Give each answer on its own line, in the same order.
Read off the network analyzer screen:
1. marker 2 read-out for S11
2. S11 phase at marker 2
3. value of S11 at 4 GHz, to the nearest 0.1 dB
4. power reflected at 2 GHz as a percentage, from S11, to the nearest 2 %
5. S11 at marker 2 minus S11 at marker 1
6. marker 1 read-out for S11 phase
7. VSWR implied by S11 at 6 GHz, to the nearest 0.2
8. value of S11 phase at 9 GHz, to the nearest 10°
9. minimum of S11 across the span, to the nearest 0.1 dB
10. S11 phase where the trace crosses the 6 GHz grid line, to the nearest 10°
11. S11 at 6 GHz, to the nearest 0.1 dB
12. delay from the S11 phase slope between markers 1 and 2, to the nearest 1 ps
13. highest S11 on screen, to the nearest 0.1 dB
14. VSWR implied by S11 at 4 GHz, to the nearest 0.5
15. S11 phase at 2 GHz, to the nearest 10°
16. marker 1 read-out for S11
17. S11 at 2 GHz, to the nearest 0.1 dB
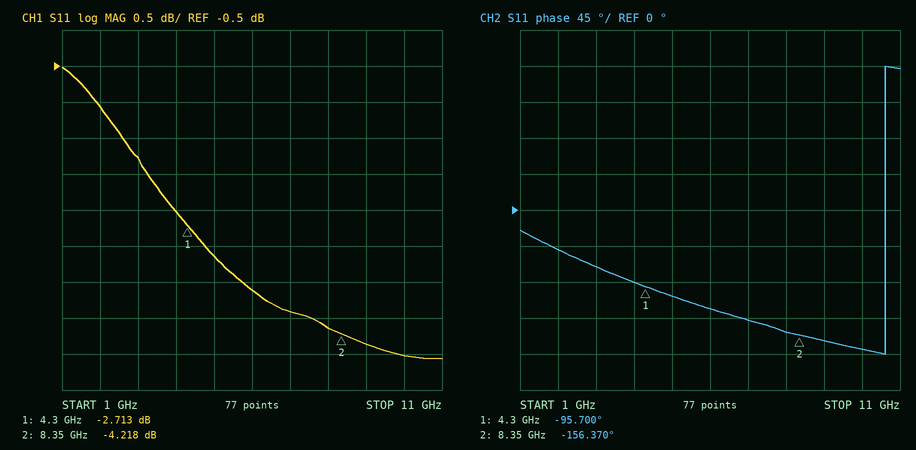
-4.218 dB
-156.370°
-2.5 dB
78 %
-1.505 dB
-95.700°
4.8
-160°
-4.6 dB
-120°
-3.6 dB
42 ps
-0.5 dB
7.0
-50°
-2.713 dB
-1.1 dB
